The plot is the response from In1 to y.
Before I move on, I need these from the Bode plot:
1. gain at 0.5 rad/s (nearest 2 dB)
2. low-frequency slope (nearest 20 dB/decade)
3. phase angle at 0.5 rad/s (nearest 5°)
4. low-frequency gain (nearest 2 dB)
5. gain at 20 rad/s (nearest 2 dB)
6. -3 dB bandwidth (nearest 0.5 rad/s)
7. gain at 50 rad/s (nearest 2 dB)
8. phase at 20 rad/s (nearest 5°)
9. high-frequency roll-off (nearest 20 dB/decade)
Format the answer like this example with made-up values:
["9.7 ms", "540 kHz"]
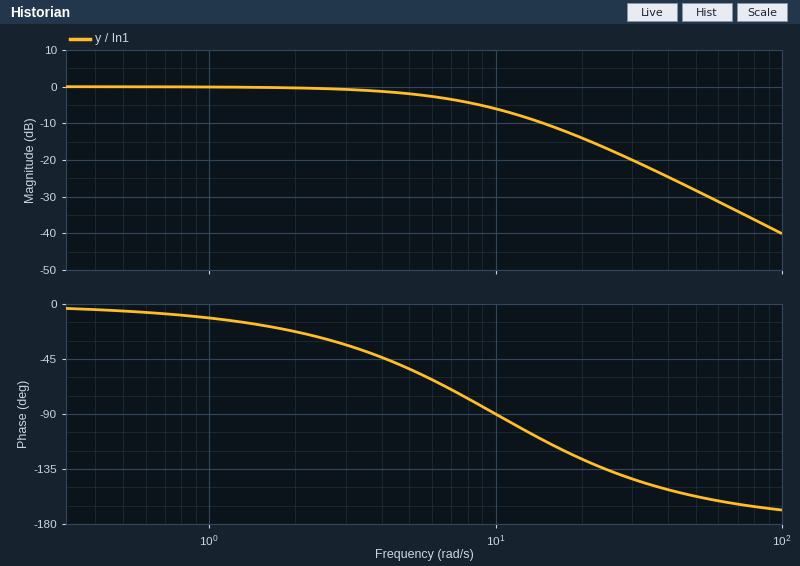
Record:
["0 dB", "0 dB/decade", "-5°", "0 dB", "-14 dB", "6.5 rad/s", "-28 dB", "-125°", "-40 dB/decade"]
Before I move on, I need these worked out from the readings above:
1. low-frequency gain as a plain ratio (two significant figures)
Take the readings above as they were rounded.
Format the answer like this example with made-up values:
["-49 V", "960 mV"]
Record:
["1.0"]
